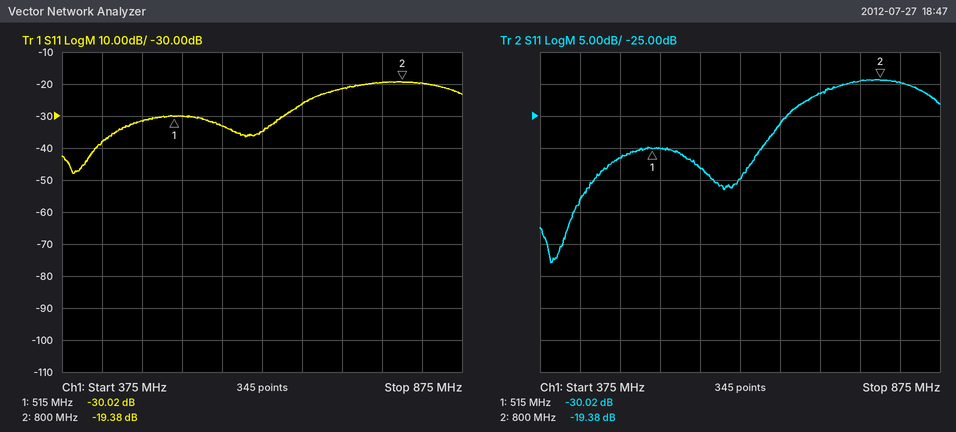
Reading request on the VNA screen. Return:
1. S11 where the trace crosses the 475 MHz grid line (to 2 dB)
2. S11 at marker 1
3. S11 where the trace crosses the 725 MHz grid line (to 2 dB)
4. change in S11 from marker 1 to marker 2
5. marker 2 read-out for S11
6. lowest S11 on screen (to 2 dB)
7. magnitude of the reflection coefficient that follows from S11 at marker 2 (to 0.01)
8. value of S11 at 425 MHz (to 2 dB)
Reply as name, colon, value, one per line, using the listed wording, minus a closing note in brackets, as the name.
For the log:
S11 where the trace crosses the 475 MHz grid line: -32 dB
S11 at marker 1: -30.02 dB
S11 where the trace crosses the 725 MHz grid line: -22 dB
change in S11 from marker 1 to marker 2: 10.64 dB
marker 2 read-out for S11: -19.38 dB
lowest S11 on screen: -48 dB
magnitude of the reflection coefficient that follows from S11 at marker 2: 0.11
value of S11 at 425 MHz: -38 dB
